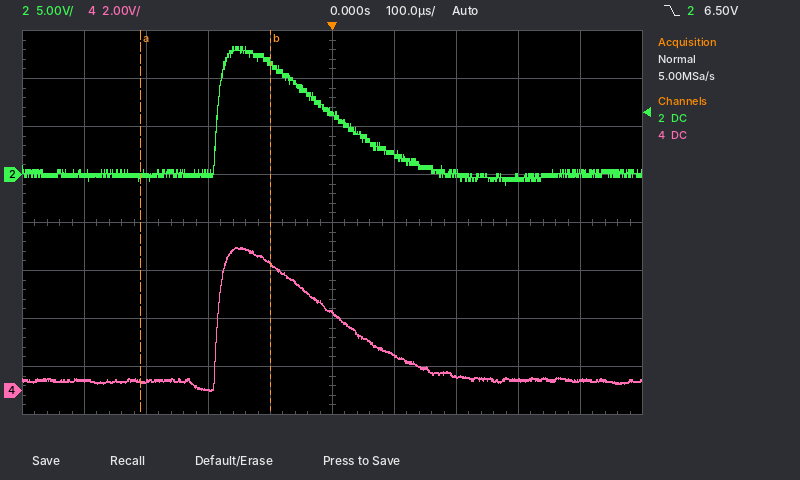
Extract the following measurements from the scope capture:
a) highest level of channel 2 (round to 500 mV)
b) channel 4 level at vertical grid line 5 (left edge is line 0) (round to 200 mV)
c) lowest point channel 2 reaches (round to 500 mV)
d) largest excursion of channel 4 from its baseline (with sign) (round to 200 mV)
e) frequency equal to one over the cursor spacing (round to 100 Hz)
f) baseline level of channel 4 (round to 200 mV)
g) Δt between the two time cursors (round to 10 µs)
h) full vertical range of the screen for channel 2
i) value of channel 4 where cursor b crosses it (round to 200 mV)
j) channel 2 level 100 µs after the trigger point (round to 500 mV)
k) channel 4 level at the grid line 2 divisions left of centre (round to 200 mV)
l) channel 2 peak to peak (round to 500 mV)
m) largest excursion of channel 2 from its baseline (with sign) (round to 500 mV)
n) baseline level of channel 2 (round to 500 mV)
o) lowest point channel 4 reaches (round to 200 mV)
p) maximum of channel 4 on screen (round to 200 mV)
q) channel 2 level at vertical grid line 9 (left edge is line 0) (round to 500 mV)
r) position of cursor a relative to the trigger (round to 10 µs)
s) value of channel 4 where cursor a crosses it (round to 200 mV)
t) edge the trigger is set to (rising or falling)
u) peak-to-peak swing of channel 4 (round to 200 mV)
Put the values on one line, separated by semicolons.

13.5 V; 3.2 V; -1.0 V; +5.6 V; 4.8 kHz; 400 mV; 210 µs; 40 V; 5.2 V; 2.0 V; 0.0 V; 14.5 V; +13.5 V; 0.0 V; 0.0 V; 6.0 V; 0.0 V; -310 µs; 400 mV; falling; 6.0 V
